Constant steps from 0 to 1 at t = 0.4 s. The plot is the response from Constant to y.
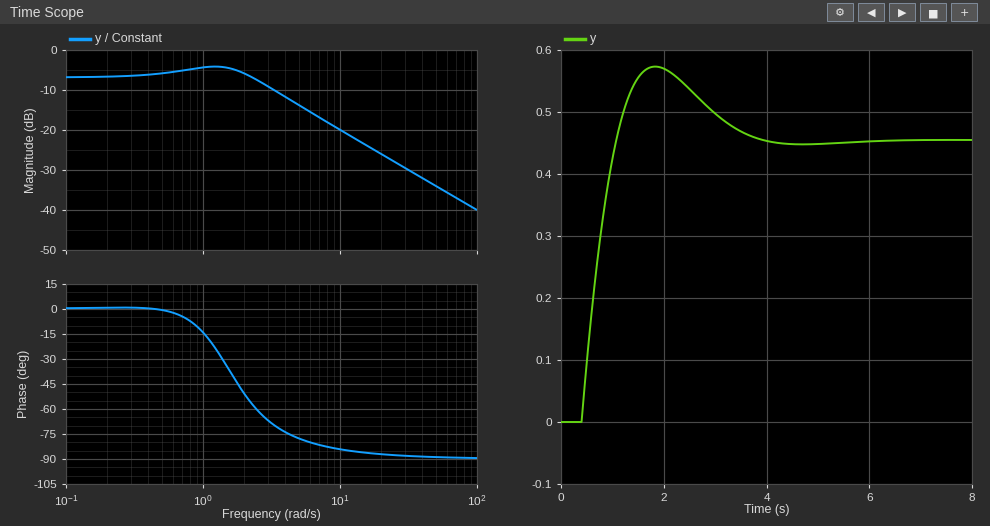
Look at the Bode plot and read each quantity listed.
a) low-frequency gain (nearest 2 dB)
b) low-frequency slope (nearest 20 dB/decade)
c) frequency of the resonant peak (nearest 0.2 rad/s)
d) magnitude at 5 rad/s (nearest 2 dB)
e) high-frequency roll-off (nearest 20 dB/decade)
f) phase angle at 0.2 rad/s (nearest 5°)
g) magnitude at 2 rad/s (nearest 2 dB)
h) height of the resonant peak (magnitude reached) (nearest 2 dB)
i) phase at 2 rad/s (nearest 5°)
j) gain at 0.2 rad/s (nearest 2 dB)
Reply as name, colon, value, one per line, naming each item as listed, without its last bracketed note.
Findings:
low-frequency gain: -6 dB
low-frequency slope: 0 dB/decade
frequency of the resonant peak: 1.2 rad/s
magnitude at 5 rad/s: -14 dB
high-frequency roll-off: -20 dB/decade
phase angle at 0.2 rad/s: 0°
magnitude at 2 rad/s: -6 dB
height of the resonant peak (magnitude reached): -4 dB
phase at 2 rad/s: -50°
gain at 0.2 rad/s: -6 dB
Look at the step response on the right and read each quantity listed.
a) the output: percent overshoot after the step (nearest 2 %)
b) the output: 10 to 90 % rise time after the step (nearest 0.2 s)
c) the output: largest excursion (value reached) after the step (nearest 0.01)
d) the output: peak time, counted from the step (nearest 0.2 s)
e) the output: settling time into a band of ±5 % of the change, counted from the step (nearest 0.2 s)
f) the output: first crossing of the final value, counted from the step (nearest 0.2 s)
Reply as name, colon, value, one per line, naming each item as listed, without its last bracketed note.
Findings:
the output: percent overshoot after the step: 26 %
the output: 10 to 90 % rise time after the step: 0.6 s
the output: largest excursion (value reached) after the step: 0.57
the output: peak time, counted from the step: 1.4 s
the output: settling time into a band of ±5 % of the change, counted from the step: 3.0 s
the output: first crossing of the final value, counted from the step: 0.6 s
